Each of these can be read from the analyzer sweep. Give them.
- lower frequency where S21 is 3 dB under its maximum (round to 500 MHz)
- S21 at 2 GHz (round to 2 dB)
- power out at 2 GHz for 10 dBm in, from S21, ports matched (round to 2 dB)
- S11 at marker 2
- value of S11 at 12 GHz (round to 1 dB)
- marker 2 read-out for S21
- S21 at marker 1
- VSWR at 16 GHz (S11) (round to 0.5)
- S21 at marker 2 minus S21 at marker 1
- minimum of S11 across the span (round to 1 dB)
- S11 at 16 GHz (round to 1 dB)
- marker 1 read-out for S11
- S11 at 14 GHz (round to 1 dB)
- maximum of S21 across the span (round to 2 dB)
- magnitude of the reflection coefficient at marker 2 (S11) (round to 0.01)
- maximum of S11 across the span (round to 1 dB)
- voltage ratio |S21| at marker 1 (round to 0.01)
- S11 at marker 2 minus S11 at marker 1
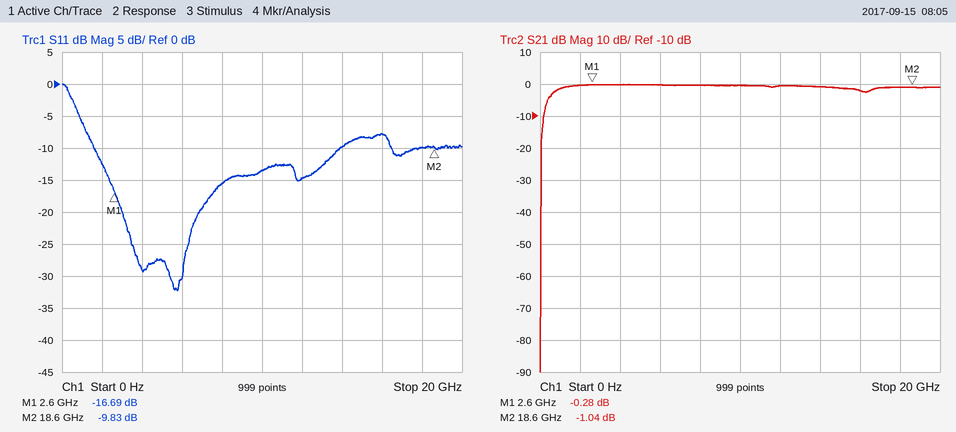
500 MHz
0 dB
10 dBm
-9.83 dB
-15 dB
-1.04 dB
-0.28 dB
2.5
-0.76 dB
-32 dB
-8 dB
-16.69 dB
-10 dB
0 dB
0.32
0 dB
0.97
6.86 dB
